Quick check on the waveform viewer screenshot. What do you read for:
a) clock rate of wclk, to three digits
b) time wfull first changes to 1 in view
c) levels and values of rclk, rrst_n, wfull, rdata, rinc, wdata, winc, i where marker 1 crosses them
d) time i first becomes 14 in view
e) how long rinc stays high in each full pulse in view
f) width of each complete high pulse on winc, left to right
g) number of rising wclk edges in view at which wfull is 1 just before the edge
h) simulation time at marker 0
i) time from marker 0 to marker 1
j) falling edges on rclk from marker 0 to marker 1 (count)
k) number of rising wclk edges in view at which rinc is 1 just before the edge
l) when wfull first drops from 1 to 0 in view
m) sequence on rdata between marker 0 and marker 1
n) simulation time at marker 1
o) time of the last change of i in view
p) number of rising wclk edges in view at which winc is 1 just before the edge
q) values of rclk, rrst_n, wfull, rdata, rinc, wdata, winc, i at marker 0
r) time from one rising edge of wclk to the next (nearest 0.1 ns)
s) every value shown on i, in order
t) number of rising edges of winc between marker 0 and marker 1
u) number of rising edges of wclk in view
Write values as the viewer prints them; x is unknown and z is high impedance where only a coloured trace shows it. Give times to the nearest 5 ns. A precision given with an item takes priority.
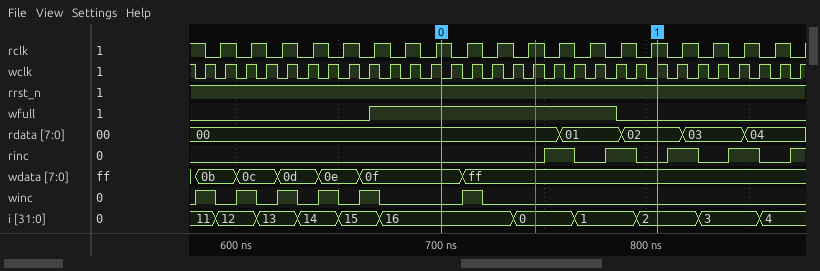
100 MHz
665 ns
rclk=1, rrst_n=1, wfull=0, rdata=02, rinc=0, wdata=ff, winc=0, i=2
630 ns
15 ns, 15 ns, 15 ns, 15 ns
10 ns, 10 ns, 10 ns, 10 ns, 10 ns, 10 ns
12
700 ns
105 ns
7
9
785 ns
00, 01, 02
805 ns
855 ns
6
rclk=1, rrst_n=1, wfull=1, rdata=00, rinc=0, wdata=0f, winc=0, i=16
10 ns
11, 12, 13, 14, 15, 16, 0, 1, 2, 3, 4
1
30
